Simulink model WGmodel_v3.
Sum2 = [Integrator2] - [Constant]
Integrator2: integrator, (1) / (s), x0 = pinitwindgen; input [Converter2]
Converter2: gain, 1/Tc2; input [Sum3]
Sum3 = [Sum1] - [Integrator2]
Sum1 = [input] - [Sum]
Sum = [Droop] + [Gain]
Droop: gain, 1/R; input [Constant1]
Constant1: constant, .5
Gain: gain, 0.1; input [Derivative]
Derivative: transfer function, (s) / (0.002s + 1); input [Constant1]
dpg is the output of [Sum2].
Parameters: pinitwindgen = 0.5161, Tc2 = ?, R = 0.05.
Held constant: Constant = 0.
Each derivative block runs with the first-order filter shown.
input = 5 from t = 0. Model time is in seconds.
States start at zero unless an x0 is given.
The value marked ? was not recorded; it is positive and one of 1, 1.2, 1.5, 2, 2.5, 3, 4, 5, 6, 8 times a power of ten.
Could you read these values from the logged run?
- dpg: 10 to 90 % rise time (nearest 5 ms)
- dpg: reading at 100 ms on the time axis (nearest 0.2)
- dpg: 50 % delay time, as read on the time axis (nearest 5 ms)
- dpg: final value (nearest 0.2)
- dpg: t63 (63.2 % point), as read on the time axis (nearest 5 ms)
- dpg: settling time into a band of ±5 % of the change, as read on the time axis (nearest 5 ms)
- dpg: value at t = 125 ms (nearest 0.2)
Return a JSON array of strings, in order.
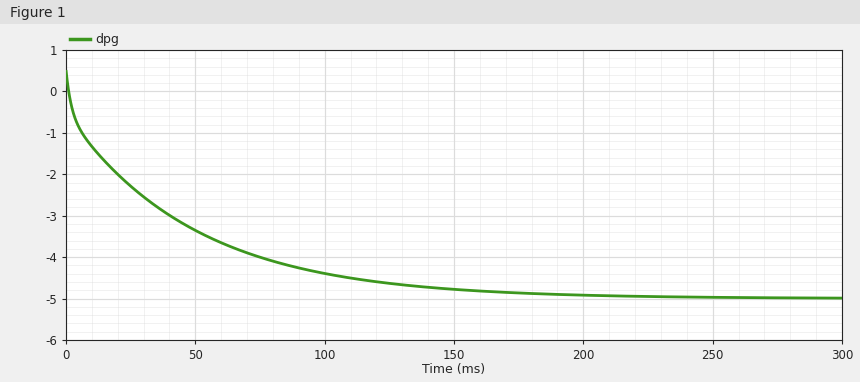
["105 ms", "-4.4", "25 ms", "-5.0", "40 ms", "140 ms", "-4.6"]
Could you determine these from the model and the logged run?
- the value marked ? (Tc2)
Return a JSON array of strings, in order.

["0.05"]
